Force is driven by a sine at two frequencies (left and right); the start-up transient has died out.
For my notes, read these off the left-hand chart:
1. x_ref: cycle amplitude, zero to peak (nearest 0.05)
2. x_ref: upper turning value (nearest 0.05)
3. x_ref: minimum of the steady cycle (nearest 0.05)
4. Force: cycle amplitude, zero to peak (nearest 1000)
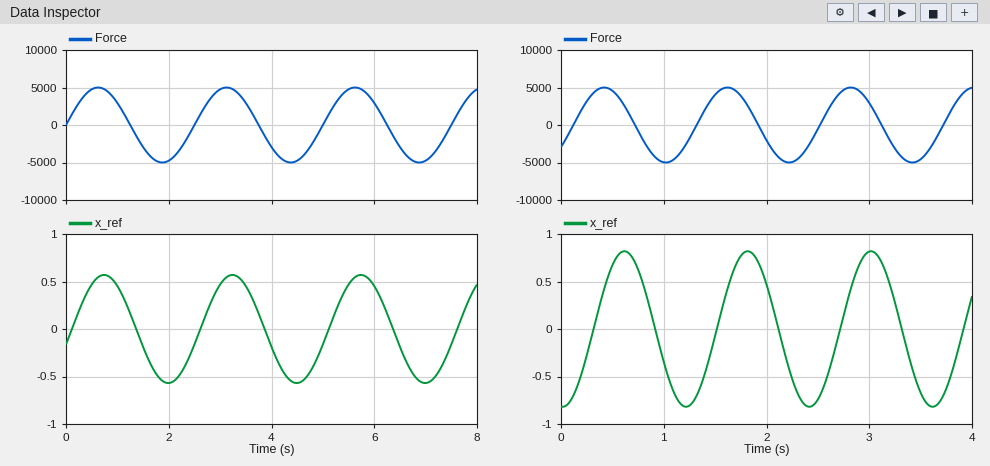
0.55
0.55
-0.55
5000
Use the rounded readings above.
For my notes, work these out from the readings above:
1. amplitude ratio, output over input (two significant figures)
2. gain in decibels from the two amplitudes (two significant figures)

0.00011
-79 dB
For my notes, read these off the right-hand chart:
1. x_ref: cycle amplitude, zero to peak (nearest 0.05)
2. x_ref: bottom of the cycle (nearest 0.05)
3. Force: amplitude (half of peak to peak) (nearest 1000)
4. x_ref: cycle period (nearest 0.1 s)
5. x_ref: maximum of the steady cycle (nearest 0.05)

0.80
-0.80
5000
1.2 s
0.80
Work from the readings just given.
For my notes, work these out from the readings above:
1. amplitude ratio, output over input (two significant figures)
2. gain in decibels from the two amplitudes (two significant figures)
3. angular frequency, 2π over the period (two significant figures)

0.00016
-76 dB
5.2 rad/s
